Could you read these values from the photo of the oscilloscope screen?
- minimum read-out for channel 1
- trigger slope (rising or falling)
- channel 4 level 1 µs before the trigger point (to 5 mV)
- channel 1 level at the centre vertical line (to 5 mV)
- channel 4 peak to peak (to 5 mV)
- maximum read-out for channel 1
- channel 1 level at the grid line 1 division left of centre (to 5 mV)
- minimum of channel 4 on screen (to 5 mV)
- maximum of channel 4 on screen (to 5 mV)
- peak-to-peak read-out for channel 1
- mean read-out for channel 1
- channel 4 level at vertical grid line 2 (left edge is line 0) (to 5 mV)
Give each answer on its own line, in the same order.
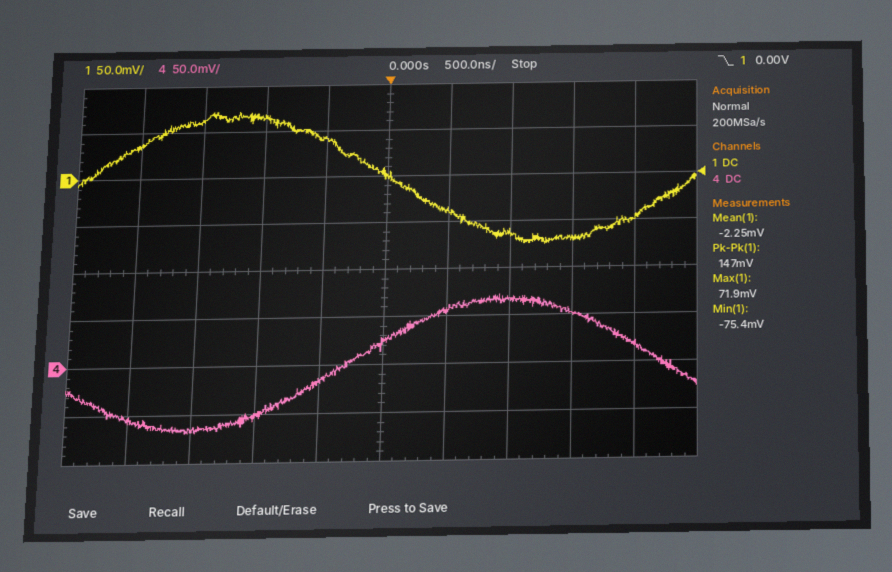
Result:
-75.4 mV
falling
-55 mV
0 mV
140 mV
71.9 mV
40 mV
-70 mV
70 mV
147 mV
-2.25 mV
-65 mV
